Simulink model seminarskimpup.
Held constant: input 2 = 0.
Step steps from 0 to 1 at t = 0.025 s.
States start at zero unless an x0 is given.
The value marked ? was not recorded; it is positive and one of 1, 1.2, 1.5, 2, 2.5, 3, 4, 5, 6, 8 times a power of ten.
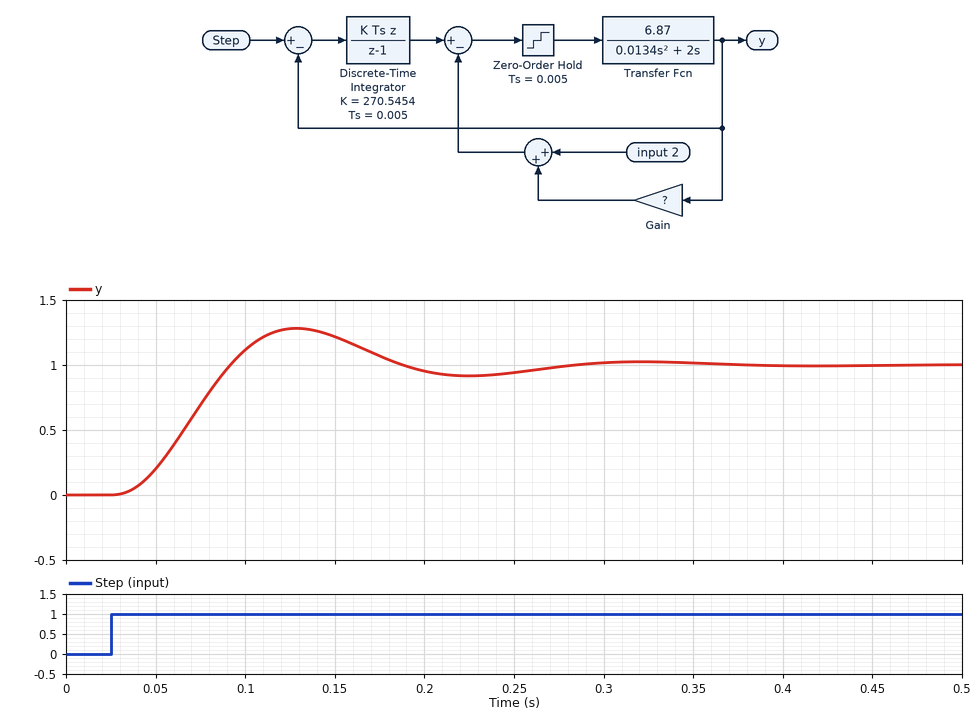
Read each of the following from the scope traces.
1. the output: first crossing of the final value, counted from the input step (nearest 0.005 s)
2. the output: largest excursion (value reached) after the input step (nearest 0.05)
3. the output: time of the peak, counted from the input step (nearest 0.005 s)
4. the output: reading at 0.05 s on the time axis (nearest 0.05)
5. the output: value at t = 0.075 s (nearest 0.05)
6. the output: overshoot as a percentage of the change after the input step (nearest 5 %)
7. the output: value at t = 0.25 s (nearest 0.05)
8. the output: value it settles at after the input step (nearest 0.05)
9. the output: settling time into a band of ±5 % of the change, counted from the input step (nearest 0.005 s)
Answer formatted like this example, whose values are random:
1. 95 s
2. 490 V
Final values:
1. 0.065 s
2. 1.30
3. 0.105 s
4. 0.20
5. 0.70
6. 30 %
7. 0.95
8. 1.00
9. 0.230 s
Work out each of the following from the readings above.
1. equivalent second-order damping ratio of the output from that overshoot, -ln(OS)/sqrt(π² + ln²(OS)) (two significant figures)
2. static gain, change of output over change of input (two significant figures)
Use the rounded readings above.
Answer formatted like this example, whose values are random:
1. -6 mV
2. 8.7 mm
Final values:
1. 0.36
2. 1.0
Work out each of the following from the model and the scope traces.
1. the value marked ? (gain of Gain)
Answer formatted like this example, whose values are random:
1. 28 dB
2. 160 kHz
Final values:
1. 8
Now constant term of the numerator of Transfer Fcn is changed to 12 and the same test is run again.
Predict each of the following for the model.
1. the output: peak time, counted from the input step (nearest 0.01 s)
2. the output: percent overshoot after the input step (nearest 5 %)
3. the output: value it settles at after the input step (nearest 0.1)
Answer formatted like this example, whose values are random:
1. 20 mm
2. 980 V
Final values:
1. 0.08 s
2. 15 %
3. 1.0
